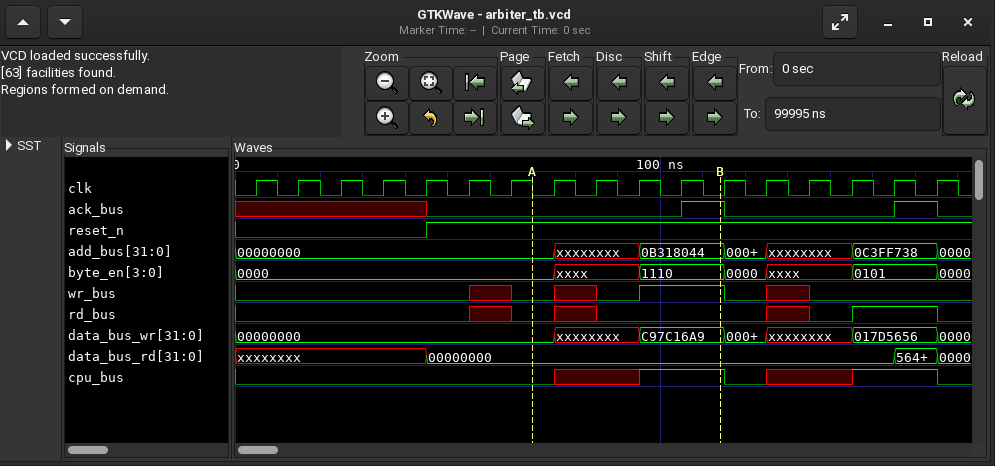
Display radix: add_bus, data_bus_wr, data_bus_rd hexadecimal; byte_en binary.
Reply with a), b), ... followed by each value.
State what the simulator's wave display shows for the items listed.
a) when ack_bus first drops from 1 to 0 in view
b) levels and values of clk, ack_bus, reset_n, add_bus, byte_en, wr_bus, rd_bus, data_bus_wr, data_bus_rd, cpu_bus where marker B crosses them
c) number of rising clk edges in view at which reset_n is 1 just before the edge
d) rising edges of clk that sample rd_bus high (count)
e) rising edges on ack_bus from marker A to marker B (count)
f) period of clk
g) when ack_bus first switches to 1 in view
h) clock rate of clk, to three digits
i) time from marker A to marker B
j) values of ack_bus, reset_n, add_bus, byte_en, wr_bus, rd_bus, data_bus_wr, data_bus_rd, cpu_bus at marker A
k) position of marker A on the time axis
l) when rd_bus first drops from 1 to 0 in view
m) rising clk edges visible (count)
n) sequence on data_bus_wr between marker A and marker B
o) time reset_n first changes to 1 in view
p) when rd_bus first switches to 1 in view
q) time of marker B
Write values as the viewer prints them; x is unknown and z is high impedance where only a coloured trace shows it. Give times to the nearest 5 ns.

a) 115 ns
b) clk=0, ack_bus=1, reset_n=1, add_bus=0B318044, byte_en=1110, wr_bus=1, rd_bus=0, data_bus_wr=C97C16A9, data_bus_rd=00000000, cpu_bus=1
c) 12
d) 2
e) 1
f) 10 ns
g) 105 ns
h) 100 MHz
i) 45 ns
j) ack_bus=0, reset_n=1, add_bus=00000000, byte_en=0000, wr_bus=0, rd_bus=0, data_bus_wr=00000000, data_bus_rd=00000000, cpu_bus=0
k) 70 ns
l) 165 ns
m) 17
n) 00000000, xxxxxxxx, C97C16A9
o) 45 ns
p) 145 ns
q) 115 ns
